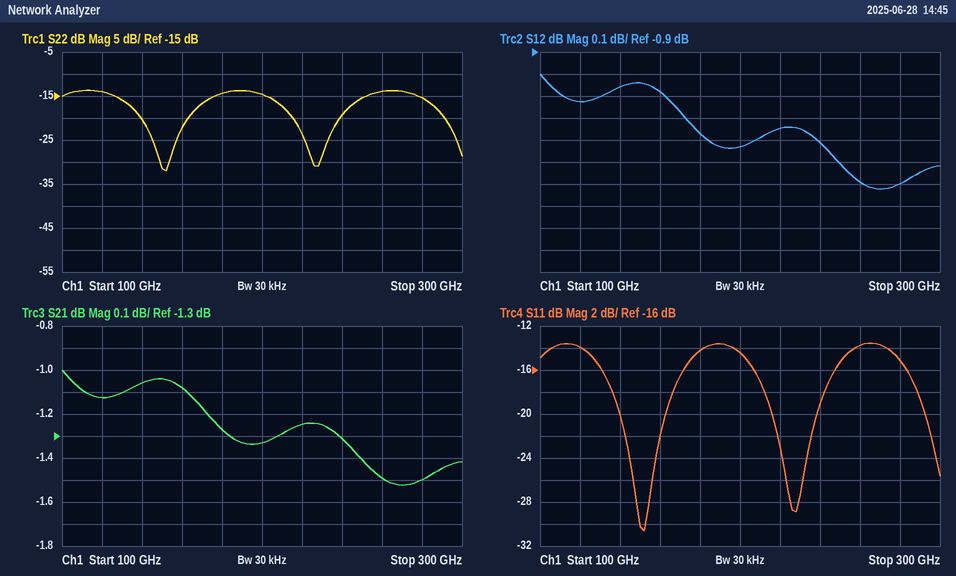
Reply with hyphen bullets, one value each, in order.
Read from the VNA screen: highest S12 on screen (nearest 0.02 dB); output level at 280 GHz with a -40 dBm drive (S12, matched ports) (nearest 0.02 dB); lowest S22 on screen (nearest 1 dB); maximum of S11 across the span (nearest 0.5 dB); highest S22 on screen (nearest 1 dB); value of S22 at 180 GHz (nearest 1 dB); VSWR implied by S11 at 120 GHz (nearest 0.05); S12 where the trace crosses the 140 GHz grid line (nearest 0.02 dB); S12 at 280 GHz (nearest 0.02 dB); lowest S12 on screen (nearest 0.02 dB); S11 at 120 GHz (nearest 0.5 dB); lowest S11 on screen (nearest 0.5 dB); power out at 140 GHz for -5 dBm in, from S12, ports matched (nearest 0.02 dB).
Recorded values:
- -1.00 dB
- -41.50 dBm
- -32 dB
- -13.5 dB
- -14 dB
- -14 dB
- 1.50
- -1.06 dB
- -1.50 dB
- -1.52 dB
- -14.0 dB
- -30.5 dB
- -6.06 dBm
